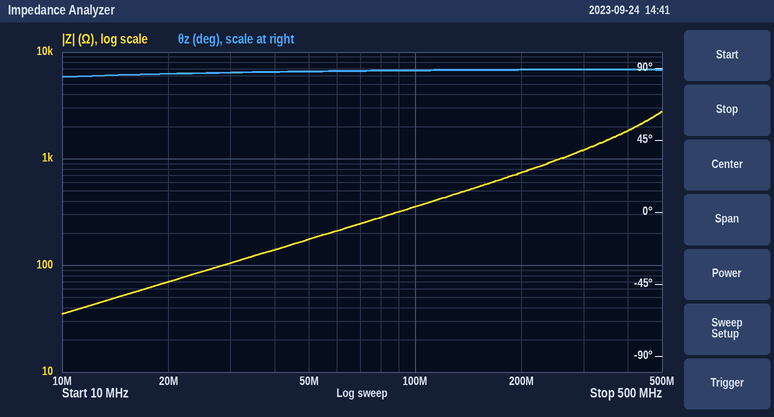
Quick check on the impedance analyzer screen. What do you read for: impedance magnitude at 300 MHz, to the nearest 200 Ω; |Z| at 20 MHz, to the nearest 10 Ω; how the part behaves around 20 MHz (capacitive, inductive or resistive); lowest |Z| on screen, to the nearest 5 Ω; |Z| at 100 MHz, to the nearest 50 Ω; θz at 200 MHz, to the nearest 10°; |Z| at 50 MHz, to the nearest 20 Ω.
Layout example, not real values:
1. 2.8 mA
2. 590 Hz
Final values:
1. 1.2 kΩ
2. 70 Ω
3. inductive
4. 35 Ω
5. 350 Ω
6. 90°
7. 180 Ω
